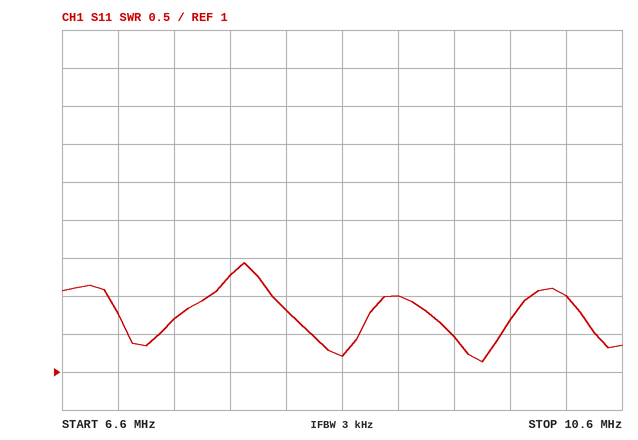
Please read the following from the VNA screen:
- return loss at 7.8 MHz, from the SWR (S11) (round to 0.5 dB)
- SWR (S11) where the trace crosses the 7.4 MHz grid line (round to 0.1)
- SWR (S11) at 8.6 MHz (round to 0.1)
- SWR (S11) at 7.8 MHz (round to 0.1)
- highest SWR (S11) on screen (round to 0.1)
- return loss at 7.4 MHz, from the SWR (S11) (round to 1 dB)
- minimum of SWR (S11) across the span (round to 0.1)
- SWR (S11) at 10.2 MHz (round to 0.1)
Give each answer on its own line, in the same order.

8.0 dB
1.7
1.2
2.3
2.4
12 dB
1.1
2.0
